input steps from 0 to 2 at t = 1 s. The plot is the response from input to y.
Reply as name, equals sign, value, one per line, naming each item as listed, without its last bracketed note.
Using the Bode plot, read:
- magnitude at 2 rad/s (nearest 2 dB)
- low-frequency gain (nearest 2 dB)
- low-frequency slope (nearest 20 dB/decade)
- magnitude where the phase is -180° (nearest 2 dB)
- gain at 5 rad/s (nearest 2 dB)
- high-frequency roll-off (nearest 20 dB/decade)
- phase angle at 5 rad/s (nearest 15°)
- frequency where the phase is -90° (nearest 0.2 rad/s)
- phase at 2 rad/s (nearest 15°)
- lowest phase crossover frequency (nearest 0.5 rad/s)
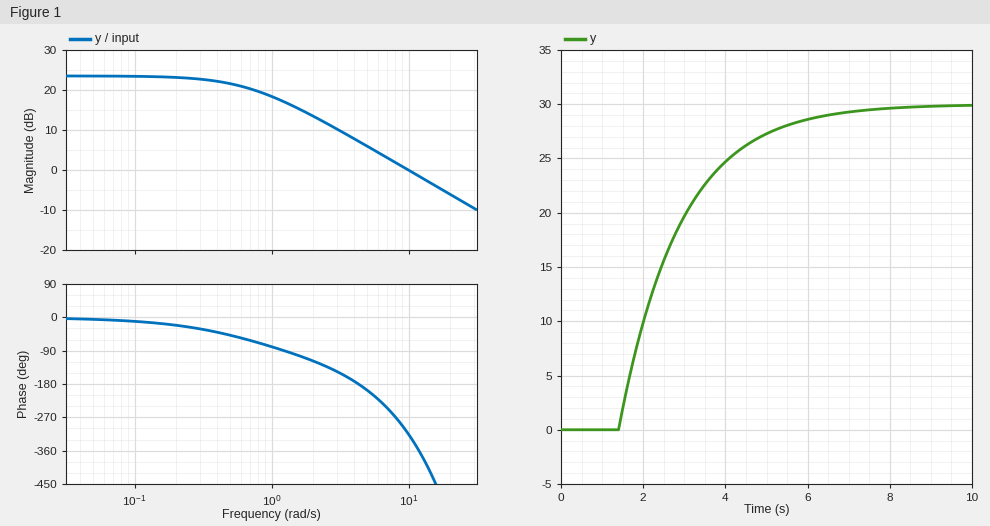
magnitude at 2 rad/s = 14 dB
low-frequency gain = 24 dB
low-frequency slope = 0 dB/decade
magnitude where the phase is -180° = 8 dB
gain at 5 rad/s = 6 dB
high-frequency roll-off = -20 dB/decade
phase angle at 5 rad/s = -195°
frequency where the phase is -90° = 1.2 rad/s
phase at 2 rad/s = -120°
lowest phase crossover frequency = 4.5 rad/s
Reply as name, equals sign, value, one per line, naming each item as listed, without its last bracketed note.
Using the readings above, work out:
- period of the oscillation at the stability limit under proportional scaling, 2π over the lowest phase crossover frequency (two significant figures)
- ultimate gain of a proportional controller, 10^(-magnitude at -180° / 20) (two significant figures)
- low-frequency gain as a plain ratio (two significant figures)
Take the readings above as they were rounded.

period of the oscillation at the stability limit under proportional scaling, 2π over the lowest phase crossover frequency = 1.4 s
ultimate gain of a proportional controller, 10^(-magnitude at -180° / 20) = 0.40
low-frequency gain as a plain ratio = 16
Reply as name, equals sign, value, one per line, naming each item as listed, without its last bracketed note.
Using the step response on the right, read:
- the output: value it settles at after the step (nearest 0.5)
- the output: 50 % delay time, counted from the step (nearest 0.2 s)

the output: value it settles at after the step = 30.0
the output: 50 % delay time, counted from the step = 1.4 s
